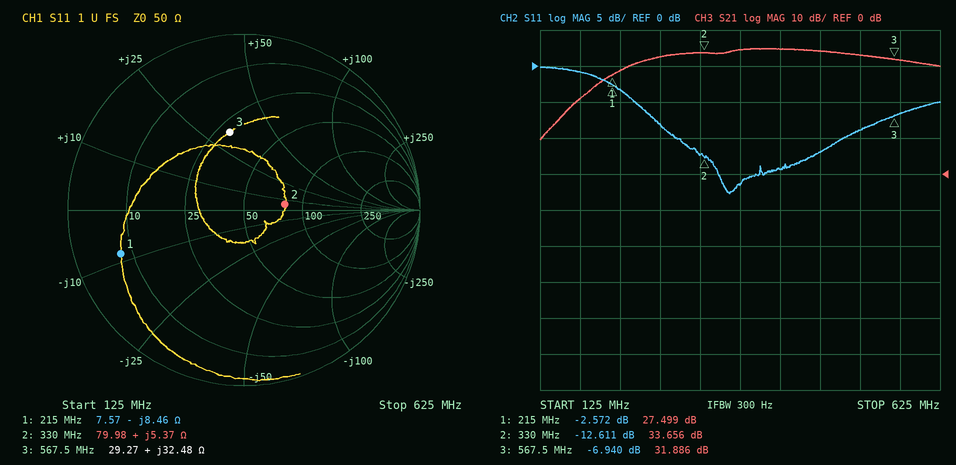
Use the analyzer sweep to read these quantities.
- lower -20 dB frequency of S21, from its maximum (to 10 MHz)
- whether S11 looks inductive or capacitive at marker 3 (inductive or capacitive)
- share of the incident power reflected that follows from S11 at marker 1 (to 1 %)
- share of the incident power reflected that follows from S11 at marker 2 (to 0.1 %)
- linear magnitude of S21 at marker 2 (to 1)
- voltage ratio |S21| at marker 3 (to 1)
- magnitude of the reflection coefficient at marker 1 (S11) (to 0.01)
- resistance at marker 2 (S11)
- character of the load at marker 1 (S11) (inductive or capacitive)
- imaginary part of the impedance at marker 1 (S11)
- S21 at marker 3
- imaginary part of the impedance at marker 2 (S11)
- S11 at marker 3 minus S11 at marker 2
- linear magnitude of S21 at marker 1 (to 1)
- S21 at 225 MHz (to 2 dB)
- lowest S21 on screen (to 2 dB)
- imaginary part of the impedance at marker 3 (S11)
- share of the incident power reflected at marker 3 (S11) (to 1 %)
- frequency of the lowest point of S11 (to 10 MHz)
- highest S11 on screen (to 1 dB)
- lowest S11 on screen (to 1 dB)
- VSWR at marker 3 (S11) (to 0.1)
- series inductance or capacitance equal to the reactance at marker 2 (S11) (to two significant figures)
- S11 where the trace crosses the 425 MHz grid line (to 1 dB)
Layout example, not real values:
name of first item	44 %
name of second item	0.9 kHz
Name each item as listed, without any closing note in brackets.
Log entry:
lower -20 dB frequency of S21, from its maximum	150 MHz
whether S11 looks inductive or capacitive at marker 3	inductive
share of the incident power reflected that follows from S11 at marker 1	55 %
share of the incident power reflected that follows from S11 at marker 2	5.5 %
linear magnitude of S21 at marker 2	48
voltage ratio |S21| at marker 3	39
magnitude of the reflection coefficient at marker 1 (S11)	0.74
resistance at marker 2	79.98 Ω
character of the load at marker 1 (S11)	capacitive
imaginary part of the impedance at marker 1	-8.46 Ω
S21 at marker 3	31.886 dB
imaginary part of the impedance at marker 2	+5.37 Ω
S11 at marker 3 minus S11 at marker 2	5.671 dB
linear magnitude of S21 at marker 1	24
S21 at 225 MHz	28 dB
lowest S21 on screen	10 dB
imaginary part of the impedance at marker 3	+32.48 Ω
share of the incident power reflected at marker 3 (S11)	20 %
frequency of the lowest point of S11	360 MHz
highest S11 on screen	0 dB
lowest S11 on screen	-18 dB
VSWR at marker 3 (S11)	2.6
series inductance or capacitance equal to the reactance at marker 2 (S11)	2.6 nH
S11 where the trace crosses the 425 MHz grid line	-14 dB
